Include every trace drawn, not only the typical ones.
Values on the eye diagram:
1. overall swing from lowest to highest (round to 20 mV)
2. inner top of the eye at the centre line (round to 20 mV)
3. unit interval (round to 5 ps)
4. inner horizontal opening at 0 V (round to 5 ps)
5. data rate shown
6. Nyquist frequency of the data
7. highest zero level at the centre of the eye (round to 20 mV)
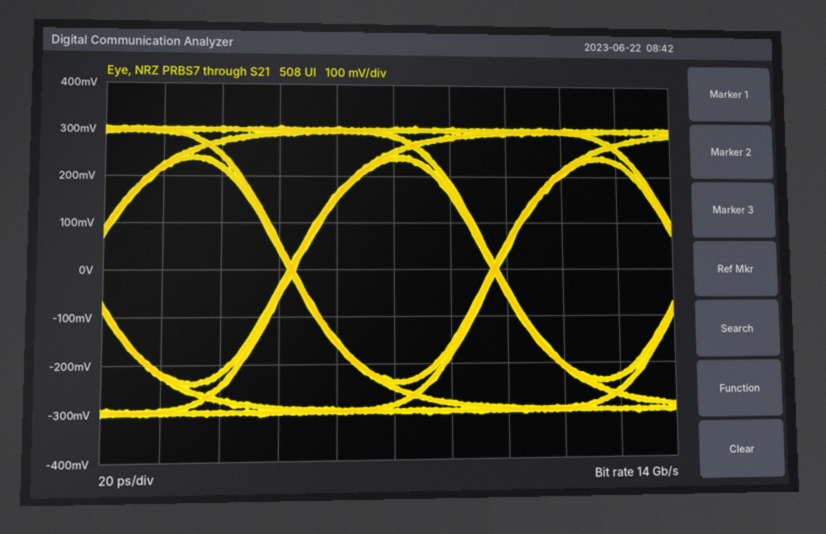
620 mV
240 mV
70 ps
70 ps
14 Gb/s
7 GHz
-240 mV
